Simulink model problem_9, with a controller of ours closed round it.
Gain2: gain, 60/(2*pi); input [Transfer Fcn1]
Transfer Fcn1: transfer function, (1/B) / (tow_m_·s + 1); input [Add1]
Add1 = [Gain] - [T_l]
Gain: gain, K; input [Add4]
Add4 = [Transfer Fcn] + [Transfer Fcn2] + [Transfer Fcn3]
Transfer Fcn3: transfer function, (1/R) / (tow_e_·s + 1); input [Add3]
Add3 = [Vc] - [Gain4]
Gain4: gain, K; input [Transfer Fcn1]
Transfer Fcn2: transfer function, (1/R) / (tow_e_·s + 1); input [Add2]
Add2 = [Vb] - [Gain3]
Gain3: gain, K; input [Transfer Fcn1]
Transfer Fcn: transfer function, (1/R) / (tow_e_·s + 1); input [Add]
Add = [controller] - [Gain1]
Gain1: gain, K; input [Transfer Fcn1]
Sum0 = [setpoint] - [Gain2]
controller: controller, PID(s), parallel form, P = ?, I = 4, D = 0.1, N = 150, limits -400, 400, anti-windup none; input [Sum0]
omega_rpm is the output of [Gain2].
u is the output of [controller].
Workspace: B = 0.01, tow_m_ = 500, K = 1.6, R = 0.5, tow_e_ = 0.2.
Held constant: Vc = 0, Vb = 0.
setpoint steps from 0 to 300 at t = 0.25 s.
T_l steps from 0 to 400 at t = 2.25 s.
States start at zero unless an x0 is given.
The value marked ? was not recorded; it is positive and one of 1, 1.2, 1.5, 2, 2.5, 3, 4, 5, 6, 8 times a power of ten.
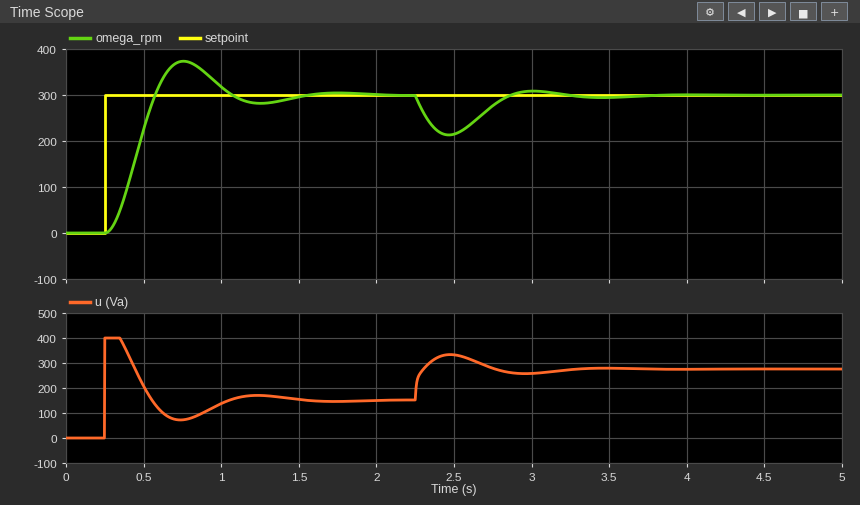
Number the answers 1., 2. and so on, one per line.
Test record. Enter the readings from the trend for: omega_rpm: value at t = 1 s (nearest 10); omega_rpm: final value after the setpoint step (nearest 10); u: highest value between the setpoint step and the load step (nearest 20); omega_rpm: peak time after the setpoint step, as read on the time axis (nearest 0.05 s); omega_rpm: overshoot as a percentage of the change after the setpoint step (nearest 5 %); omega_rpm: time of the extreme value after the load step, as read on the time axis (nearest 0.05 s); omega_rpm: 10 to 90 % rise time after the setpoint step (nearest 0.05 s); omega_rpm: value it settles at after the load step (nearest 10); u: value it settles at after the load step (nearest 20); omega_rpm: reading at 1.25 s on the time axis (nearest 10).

1. 320
2. 300
3. 400
4. 0.75 s
5. 25 %
6. 2.45 s
7. 0.20 s
8. 300
9. 280
10. 280
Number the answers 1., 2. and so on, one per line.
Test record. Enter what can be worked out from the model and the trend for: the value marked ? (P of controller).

1. 1.5
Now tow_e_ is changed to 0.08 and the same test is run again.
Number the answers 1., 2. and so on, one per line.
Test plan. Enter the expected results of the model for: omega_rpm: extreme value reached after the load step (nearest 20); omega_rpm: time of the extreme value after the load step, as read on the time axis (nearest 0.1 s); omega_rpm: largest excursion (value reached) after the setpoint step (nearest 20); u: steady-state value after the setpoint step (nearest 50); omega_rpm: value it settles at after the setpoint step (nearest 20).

1. 240
2. 2.4 s
3. 320
4. 150
5. 300
